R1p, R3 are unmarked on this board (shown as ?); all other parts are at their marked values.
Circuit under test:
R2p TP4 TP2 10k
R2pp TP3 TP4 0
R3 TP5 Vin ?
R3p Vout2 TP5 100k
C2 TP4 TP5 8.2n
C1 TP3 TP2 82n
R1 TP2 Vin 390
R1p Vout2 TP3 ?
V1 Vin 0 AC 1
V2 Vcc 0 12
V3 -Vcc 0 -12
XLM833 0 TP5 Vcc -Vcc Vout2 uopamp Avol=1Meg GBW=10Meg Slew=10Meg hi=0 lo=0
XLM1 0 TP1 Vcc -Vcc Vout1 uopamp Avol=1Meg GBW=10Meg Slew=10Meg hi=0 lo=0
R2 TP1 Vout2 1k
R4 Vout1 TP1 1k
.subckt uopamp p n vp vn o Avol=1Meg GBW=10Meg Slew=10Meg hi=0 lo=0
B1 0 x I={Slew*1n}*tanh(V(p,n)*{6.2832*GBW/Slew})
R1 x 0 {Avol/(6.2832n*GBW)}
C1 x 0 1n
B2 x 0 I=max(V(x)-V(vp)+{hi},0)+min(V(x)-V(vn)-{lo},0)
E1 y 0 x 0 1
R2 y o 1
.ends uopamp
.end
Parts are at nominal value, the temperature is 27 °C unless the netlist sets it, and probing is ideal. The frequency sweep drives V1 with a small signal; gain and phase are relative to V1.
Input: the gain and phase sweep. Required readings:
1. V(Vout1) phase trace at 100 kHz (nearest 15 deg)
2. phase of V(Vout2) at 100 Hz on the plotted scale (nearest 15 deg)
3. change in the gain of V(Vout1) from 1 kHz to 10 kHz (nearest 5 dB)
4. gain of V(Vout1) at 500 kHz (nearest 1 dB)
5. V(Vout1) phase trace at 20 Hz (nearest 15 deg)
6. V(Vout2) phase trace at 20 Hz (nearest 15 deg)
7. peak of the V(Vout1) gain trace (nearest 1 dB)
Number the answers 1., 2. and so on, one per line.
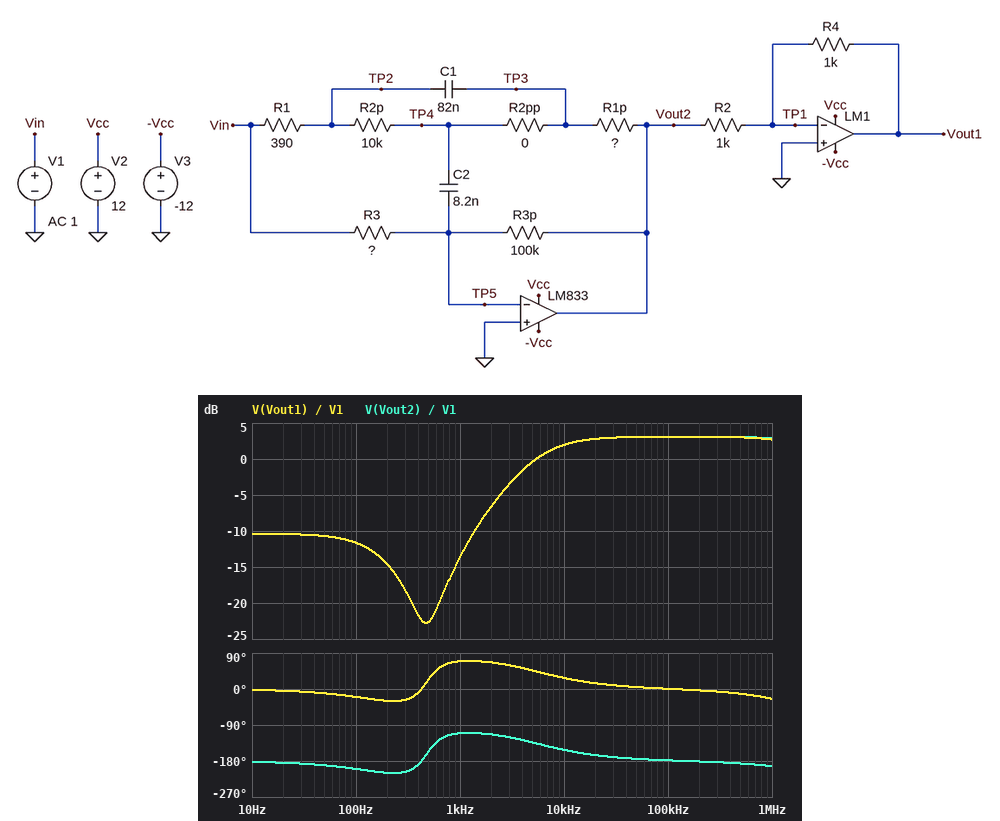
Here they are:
1. 0 deg
2. -195 deg
3. 15 dB
4. 3 dB
5. 0 deg
6. -180 deg
7. 3 dB
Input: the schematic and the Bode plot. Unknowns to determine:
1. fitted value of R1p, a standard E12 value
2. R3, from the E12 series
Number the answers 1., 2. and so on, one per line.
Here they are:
1. 560 Ω
2. 330 kΩ
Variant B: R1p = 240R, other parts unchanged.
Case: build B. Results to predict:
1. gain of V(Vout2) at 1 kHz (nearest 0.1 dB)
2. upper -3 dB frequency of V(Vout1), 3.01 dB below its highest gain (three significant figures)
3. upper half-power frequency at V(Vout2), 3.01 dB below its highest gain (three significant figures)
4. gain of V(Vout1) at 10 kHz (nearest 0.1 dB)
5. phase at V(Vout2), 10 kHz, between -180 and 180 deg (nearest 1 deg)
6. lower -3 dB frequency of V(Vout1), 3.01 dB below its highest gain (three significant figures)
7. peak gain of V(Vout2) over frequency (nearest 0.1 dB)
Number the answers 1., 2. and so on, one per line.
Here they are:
1. -23.4 dB
2. 3.56 MHz
3. 6.20 MHz
4. -5.3 dB
5. -153 deg
6. 5.45 kHz
7. -4.2 dB
